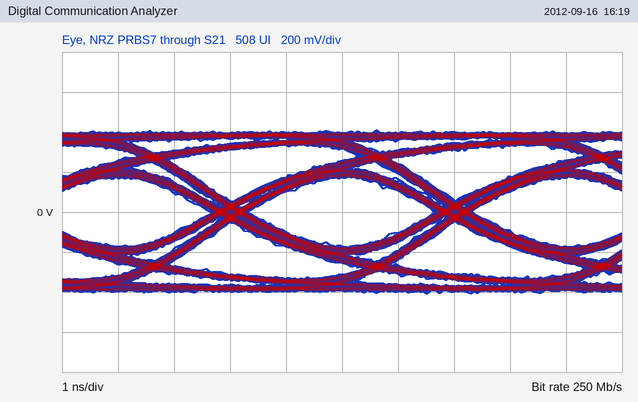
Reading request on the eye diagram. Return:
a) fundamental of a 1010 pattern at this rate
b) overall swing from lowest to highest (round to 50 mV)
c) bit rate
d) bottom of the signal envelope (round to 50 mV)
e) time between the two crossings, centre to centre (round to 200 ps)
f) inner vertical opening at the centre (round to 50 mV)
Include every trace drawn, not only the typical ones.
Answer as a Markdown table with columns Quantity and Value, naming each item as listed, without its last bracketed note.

| Quantity | Value |
|---|---|
| fundamental of a 1010 pattern at this rate | 125 MHz |
| overall swing from lowest to highest | 800 mV |
| bit rate | 250 Mb/s |
| bottom of the signal envelope | -400 mV |
| time between the two crossings, centre to centre | 4.0 ns |
| inner vertical opening at the centre | 350 mV |
